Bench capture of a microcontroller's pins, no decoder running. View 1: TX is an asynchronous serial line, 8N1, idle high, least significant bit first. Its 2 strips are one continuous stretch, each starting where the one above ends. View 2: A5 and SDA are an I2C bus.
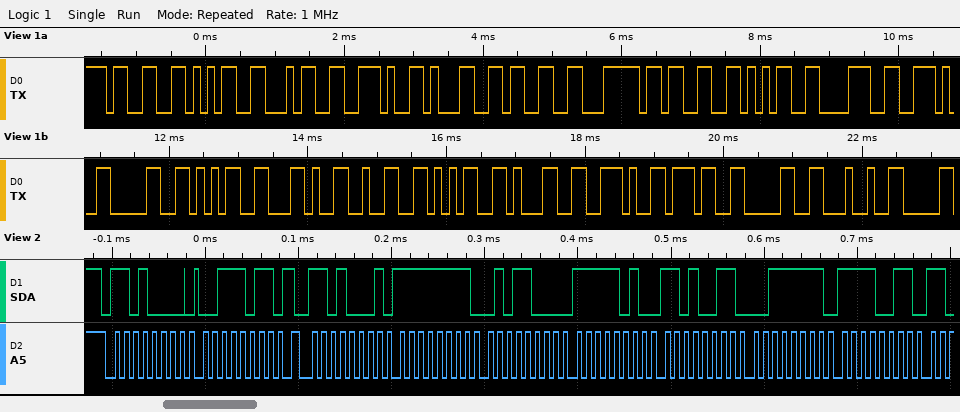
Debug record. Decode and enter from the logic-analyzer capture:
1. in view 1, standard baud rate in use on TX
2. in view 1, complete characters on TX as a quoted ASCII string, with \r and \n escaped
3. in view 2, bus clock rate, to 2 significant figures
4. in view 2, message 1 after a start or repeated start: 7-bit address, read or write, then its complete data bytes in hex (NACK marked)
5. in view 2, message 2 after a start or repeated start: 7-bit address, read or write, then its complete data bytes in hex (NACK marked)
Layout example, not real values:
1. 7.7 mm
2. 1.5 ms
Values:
1. 9600 baud
2. "354.13|358.05,251.70$"
3. 100 kHz
4. 0x68 write: 3B
5. 0x68 read: FF 58 FA D3 3F F3
